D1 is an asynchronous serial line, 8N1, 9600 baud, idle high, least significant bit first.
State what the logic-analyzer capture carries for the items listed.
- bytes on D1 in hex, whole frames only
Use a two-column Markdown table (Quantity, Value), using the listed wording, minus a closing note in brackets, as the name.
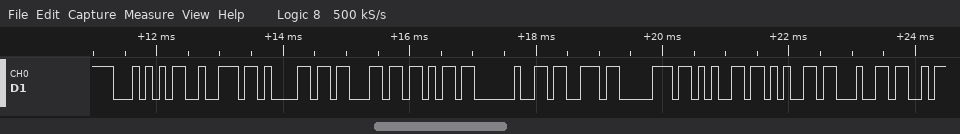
| Quantity | Value |
|---|---|
| bytes on D1 in hex, whole frames only | 0x54 0x72 0x61 0x63 0x6B 0x20 0x73 0x70 0x65 0x65 0x64 |
